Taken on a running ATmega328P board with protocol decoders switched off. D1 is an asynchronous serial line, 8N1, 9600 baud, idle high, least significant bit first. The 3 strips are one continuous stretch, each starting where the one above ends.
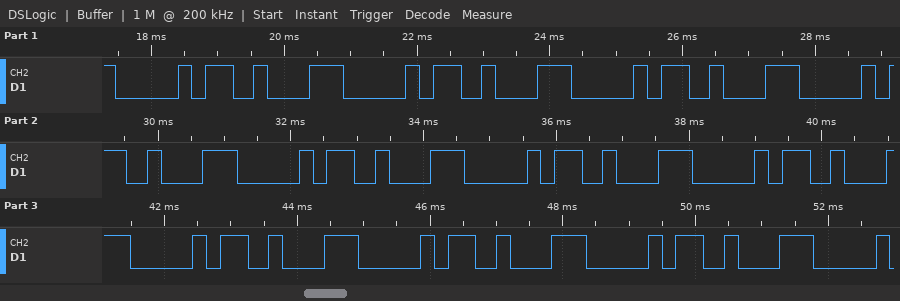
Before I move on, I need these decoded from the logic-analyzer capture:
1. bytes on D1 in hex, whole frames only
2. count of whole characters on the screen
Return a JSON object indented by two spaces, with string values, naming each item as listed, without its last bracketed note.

{
  "bytes on D1 in hex, whole frames only": "00 1E E0 00 1E E0 00 1E E0 00 1E E0 00 1E E0 00 1E E0 00 1E E0 00 1E E0 00 1E E0 00 1E E0 00",
  "count of whole characters on the screen": "31"
}
